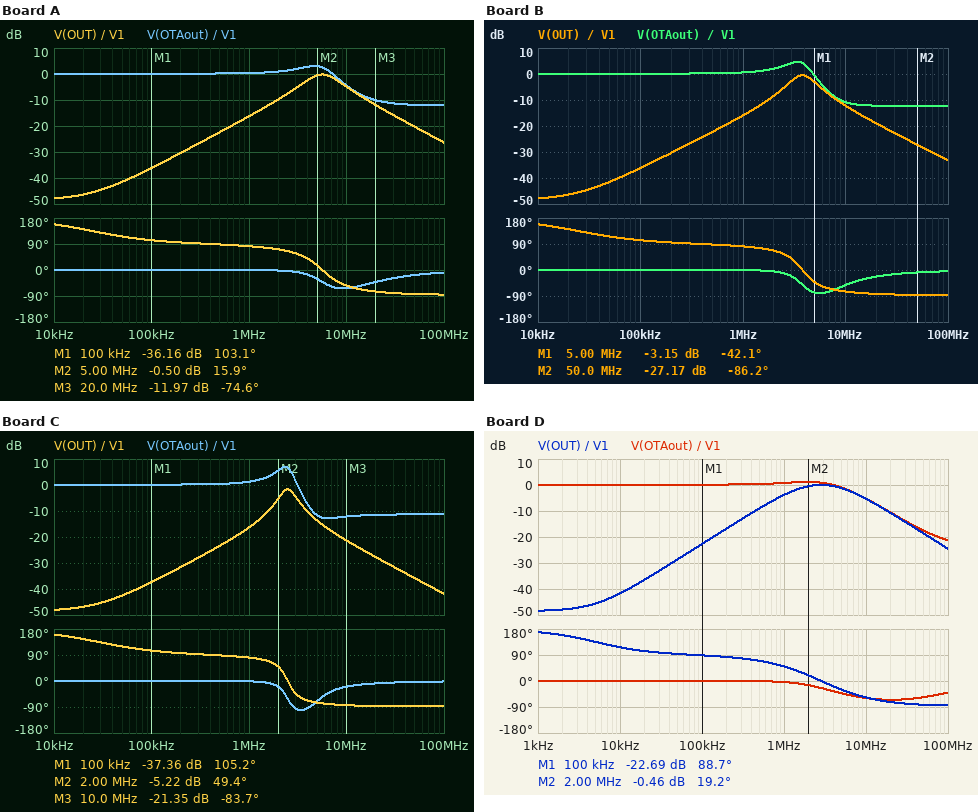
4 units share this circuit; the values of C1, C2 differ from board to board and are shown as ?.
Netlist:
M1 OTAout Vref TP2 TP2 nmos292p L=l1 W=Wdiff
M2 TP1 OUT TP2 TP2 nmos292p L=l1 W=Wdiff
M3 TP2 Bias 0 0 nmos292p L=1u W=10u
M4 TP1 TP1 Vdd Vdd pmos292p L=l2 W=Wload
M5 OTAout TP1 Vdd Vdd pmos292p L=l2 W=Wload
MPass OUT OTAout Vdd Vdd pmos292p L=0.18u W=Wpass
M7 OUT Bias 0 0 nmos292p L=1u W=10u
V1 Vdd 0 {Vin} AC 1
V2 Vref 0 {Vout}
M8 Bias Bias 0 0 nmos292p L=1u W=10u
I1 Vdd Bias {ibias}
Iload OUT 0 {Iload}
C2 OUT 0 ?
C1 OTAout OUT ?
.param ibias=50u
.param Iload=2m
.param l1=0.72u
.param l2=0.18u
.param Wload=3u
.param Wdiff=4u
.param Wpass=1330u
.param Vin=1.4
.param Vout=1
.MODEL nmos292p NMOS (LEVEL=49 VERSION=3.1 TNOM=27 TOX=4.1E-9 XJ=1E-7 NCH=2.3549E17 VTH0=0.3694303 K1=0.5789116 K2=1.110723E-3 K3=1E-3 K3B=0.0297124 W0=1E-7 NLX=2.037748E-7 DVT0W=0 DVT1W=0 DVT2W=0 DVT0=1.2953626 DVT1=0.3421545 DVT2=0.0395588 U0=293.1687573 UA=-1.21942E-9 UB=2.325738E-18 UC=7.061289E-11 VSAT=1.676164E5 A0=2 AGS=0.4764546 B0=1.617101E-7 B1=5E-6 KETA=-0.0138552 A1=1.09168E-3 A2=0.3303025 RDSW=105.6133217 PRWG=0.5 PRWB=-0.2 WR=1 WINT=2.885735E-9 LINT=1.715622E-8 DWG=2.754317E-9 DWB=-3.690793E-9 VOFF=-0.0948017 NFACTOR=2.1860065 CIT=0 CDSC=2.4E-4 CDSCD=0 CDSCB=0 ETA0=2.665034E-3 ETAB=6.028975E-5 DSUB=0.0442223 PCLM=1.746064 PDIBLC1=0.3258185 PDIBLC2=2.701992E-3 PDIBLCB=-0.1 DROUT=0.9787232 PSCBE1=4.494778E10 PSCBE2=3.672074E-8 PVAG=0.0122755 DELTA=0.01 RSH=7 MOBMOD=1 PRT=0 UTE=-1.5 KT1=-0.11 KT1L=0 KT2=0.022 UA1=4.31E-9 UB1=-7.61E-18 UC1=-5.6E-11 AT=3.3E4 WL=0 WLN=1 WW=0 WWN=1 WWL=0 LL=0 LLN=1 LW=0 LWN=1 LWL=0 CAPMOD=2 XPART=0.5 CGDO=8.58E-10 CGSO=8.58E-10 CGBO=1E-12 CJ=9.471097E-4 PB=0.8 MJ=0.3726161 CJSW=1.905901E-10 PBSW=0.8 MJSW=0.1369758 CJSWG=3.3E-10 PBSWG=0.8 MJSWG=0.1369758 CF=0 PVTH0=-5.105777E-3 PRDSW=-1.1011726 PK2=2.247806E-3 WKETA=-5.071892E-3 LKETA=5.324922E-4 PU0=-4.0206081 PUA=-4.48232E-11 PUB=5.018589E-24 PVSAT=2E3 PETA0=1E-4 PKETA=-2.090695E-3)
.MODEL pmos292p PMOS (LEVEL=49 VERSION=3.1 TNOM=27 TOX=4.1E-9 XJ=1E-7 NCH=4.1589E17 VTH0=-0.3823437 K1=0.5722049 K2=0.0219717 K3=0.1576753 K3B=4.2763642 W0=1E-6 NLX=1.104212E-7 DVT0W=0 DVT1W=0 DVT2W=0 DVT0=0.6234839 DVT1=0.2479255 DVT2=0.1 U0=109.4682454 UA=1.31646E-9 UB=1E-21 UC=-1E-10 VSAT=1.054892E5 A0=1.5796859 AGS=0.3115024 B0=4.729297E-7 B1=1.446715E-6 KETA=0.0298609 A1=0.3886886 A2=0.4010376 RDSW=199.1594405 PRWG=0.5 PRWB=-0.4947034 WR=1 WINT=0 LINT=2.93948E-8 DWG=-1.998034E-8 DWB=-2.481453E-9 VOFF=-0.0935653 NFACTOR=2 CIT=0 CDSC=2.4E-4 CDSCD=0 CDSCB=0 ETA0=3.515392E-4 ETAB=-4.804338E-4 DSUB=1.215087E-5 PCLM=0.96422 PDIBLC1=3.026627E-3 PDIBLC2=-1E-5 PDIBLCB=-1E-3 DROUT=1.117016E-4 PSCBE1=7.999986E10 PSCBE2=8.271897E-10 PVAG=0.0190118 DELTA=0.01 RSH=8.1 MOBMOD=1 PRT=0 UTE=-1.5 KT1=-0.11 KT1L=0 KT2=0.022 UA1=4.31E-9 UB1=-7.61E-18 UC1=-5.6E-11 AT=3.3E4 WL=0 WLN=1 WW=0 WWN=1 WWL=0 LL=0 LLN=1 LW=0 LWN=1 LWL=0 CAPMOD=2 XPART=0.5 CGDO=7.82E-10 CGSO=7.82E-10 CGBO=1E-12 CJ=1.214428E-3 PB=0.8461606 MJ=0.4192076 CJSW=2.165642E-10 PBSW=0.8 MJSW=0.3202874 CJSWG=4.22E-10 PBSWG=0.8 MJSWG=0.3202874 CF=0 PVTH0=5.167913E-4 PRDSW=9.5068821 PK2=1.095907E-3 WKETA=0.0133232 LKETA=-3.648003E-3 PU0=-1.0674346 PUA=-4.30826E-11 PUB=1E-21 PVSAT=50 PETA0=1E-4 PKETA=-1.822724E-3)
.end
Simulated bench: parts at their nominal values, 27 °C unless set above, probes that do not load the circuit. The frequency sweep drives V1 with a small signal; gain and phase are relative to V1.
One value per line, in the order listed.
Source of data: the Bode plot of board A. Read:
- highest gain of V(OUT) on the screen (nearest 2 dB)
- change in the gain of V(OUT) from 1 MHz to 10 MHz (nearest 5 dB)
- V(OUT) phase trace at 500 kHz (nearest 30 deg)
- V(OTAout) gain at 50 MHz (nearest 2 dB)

0 dB
10 dB
90 deg
-12 dB
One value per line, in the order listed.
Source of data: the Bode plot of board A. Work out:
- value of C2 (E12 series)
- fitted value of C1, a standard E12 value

680 pF
4.7 pF
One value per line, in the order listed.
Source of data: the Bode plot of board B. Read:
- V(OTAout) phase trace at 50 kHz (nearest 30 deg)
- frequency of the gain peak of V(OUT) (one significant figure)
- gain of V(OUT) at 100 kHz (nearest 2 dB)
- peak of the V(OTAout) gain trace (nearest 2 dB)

0 deg
4 MHz
-36 dB
4 dB
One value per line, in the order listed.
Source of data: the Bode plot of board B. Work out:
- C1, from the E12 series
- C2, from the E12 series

4.7 pF
1.5 nF
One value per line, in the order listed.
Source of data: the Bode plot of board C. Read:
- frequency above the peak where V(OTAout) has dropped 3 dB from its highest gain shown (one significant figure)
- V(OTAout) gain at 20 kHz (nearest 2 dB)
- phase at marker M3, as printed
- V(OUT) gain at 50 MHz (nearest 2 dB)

3 MHz
0 dB
-83.7 deg
-36 dB
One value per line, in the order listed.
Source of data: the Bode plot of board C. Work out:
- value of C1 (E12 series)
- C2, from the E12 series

3.9 pF
3.9 nF
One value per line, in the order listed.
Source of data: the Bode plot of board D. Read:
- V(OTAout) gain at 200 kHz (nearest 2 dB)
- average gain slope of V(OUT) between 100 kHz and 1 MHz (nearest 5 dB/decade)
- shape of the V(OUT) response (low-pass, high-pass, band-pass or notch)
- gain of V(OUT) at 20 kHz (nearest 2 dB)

0 dB
20 dB/decade
band-pass
-36 dB
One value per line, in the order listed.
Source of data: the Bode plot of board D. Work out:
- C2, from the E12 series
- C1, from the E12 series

680 pF
27 pF
